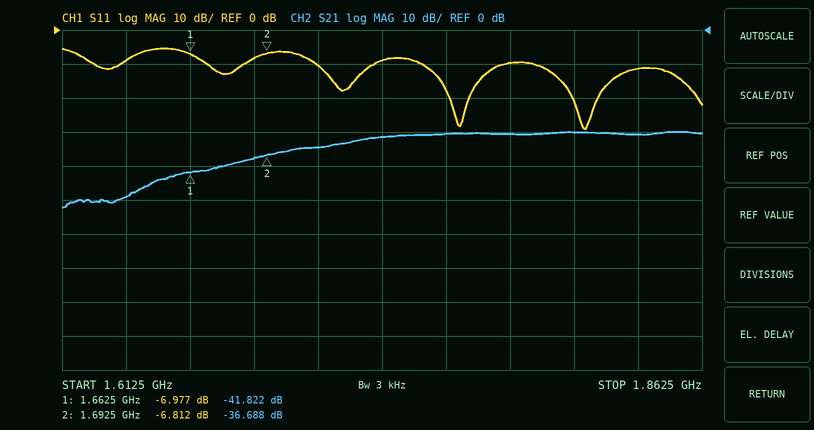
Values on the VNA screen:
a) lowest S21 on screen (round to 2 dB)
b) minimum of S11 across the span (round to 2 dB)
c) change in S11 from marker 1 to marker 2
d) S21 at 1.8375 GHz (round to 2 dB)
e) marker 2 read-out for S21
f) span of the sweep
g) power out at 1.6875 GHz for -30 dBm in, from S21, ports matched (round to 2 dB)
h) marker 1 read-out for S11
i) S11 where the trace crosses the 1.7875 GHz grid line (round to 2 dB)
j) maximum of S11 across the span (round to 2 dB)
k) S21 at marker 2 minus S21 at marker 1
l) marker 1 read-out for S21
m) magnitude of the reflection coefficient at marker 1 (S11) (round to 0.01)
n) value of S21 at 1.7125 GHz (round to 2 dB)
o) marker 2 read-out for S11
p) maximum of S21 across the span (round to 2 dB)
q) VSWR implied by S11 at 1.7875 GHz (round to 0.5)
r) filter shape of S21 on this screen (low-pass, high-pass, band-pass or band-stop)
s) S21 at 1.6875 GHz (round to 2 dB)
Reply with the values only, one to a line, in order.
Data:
-52 dB
-30 dB
0.165 dB
-30 dB
-36.688 dB
250 MHz
-68 dBm
-6.977 dB
-10 dB
-6 dB
5.134 dB
-41.822 dB
0.45
-34 dB
-6.812 dB
-30 dB
2.0
high-pass
-38 dB
